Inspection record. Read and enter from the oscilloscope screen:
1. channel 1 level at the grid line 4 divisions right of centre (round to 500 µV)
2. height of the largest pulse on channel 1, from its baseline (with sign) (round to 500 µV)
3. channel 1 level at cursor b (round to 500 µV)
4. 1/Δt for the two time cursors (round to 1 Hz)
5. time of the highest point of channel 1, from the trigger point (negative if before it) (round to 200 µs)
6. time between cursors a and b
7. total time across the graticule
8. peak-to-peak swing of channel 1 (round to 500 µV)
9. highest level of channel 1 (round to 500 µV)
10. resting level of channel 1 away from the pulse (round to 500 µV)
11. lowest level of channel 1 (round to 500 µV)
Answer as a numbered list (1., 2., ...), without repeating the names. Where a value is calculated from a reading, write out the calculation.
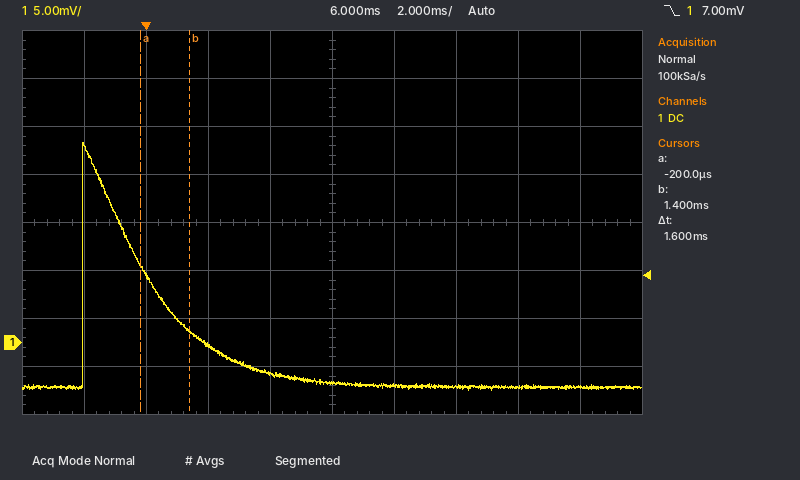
1. -4.5 mV
2. 21.0 mV − (-4.5 mV) = +25.5 mV
3. 1.0 mV
4. 1 / 1.6 ms ≈ 625 Hz
5. -2.0 ms
6. 1.6 ms
7. 20 ms
8. 21.0 mV − (-5.0 mV) = 26.0 mV
9. 21.0 mV
10. -4.5 mV
11. -5.0 mV
